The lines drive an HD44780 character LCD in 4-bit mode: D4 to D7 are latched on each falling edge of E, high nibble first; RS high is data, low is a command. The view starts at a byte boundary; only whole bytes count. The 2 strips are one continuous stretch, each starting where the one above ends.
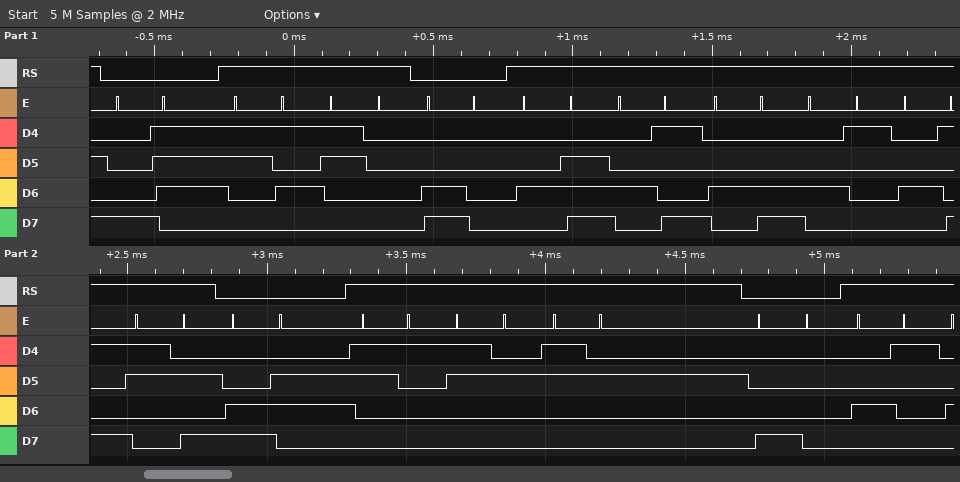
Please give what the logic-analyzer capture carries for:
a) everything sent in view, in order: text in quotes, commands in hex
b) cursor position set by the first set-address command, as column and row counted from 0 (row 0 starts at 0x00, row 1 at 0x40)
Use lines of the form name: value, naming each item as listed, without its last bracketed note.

everything sent in view, in order: text in quotes, commands in hex: 0x87 "50" 0xC0 "NILAI:" 0xC6 "122" 0x80 "A"
cursor position set by the first set-address command, as column and row counted from 0: column 7, row 0
